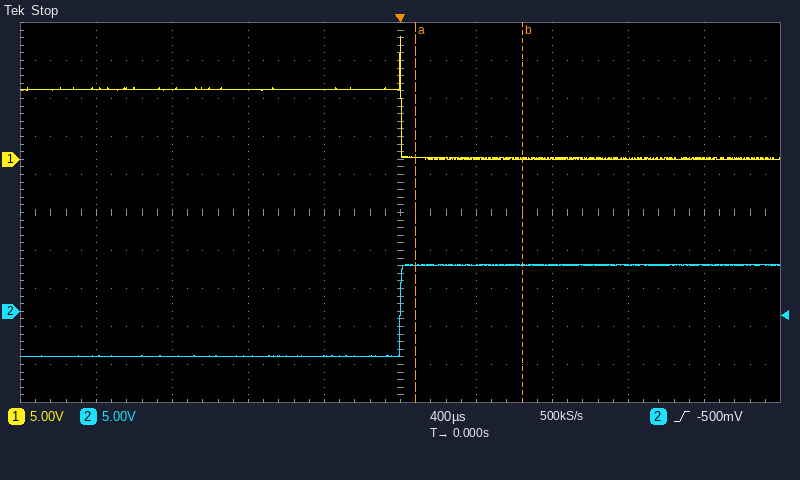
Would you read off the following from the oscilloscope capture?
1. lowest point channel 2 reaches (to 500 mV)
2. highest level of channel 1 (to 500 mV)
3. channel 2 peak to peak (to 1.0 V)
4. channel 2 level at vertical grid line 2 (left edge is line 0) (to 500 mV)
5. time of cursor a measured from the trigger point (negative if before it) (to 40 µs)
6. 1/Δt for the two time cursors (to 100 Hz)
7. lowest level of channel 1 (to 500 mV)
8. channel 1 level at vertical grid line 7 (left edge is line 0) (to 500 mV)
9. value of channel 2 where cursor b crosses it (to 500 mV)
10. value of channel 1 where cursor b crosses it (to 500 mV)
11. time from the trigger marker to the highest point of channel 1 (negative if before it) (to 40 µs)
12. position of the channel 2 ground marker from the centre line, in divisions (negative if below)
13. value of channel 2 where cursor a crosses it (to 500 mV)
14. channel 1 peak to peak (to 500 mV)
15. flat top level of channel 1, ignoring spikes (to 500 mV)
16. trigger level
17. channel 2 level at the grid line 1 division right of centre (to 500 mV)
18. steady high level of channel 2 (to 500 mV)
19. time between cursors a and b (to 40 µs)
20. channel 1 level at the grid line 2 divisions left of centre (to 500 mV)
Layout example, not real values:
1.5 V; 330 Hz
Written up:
-6.0 V; 16.0 V; 12.0 V; -6.0 V; +80 µs; 1.8 kHz; 0.0 V; 0.0 V; 6.0 V; 0.0 V; 0 µs; -2.6 div; 6.0 V; 16.0 V; 9.0 V; -500 mV; 6.0 V; 6.0 V; 560 µs; 9.0 V
